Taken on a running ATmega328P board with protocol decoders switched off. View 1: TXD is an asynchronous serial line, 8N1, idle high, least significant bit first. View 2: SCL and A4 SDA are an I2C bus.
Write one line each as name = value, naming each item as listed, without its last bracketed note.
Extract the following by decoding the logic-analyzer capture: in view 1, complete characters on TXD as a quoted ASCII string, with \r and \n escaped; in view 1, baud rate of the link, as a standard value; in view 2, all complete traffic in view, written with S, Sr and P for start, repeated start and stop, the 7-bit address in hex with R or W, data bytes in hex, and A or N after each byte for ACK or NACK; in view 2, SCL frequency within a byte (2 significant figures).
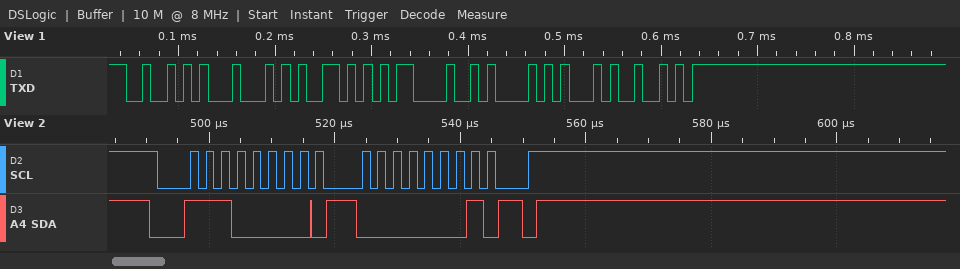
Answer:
in view 1, complete characters on TXD as a quoted ASCII string, with \r and \n escaped = "RDY\r\nER"
in view 1, baud rate of the link, as a standard value = 115200 baud
in view 2, all complete traffic in view, written with S, Sr and P for start, repeated start and stop, the 7-bit address in hex with R or W, data bytes in hex, and A or N after each byte for ACK or NACK = S 70W A 01 A P
in view 2, SCL frequency within a byte = 400 kHz
